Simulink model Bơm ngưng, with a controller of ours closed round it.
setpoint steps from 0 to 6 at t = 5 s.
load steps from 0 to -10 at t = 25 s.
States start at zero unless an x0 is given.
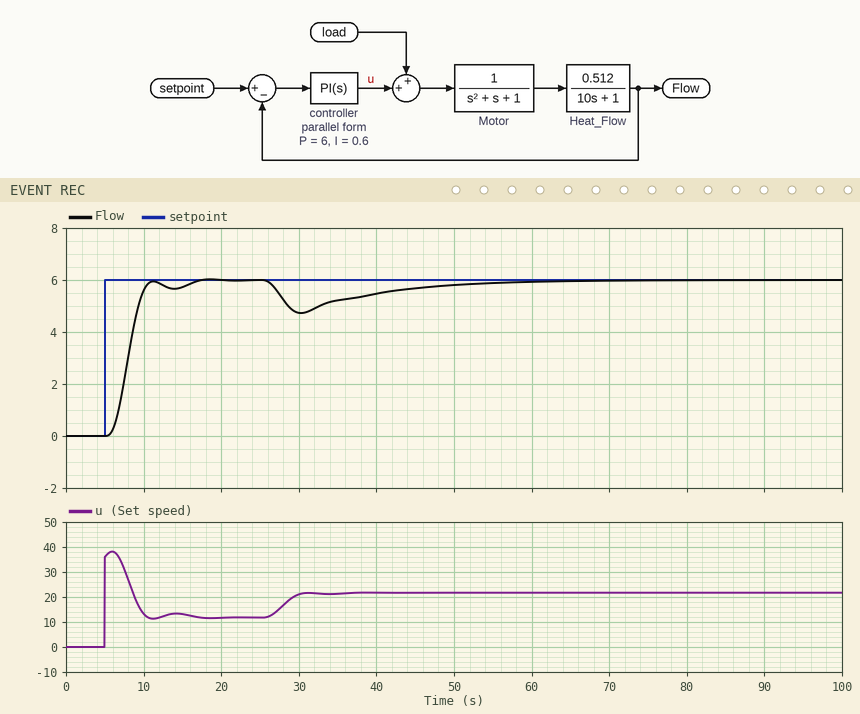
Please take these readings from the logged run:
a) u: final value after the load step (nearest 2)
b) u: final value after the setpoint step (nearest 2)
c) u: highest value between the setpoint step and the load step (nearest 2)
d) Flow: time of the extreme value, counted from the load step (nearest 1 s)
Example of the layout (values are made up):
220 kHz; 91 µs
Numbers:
22; 12; 38; 5 s
